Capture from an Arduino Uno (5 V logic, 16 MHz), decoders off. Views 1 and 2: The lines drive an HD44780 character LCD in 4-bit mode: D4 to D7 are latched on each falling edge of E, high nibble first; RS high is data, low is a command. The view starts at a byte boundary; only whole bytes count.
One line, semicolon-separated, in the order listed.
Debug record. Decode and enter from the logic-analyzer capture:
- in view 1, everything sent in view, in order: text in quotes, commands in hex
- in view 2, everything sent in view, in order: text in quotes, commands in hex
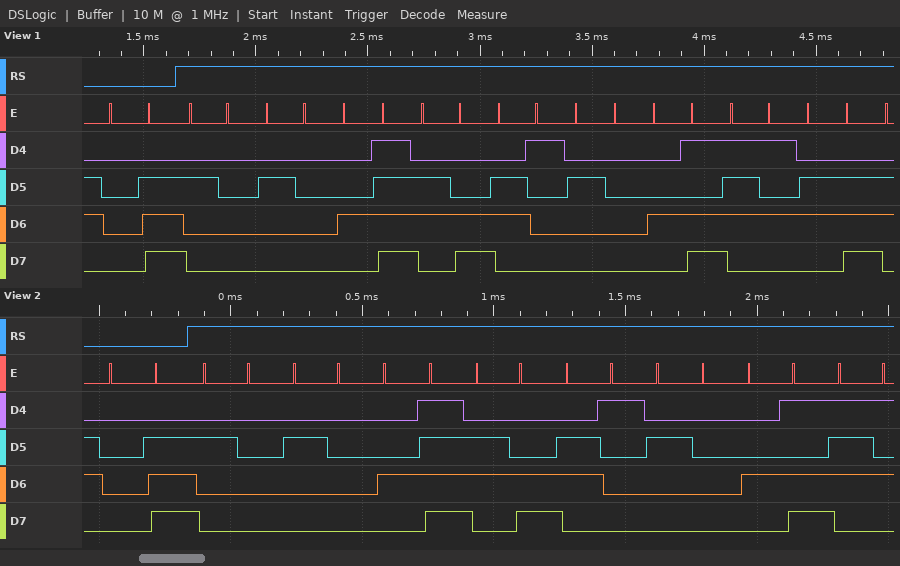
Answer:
0x0E "  Ola Mun"; 0x0E "  Ola Mu"
